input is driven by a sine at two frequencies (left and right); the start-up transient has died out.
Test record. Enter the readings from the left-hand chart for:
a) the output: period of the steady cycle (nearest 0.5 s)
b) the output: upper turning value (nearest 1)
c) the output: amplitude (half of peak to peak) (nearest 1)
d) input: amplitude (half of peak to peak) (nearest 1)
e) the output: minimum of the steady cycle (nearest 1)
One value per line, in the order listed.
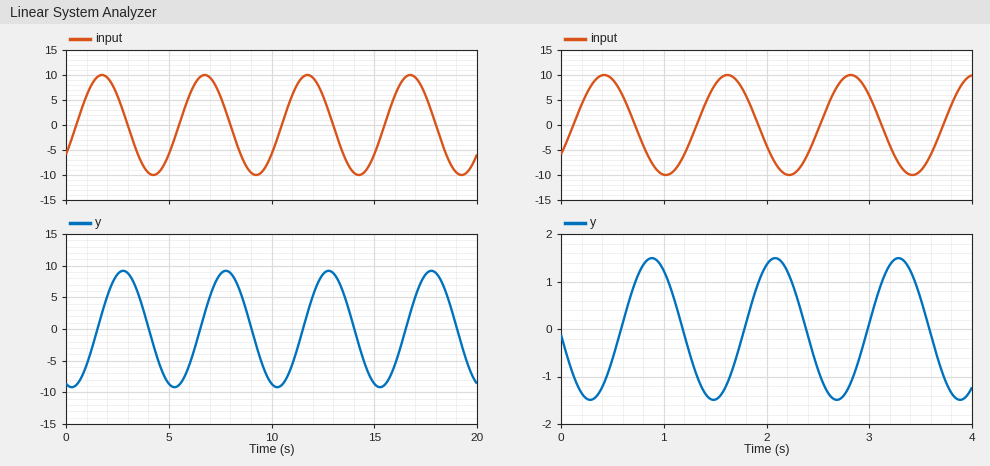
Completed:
5.0 s
9
9
10
-9
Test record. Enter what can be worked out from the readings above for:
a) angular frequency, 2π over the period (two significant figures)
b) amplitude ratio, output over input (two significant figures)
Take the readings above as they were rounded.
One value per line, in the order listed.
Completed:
1.3 rad/s
0.90
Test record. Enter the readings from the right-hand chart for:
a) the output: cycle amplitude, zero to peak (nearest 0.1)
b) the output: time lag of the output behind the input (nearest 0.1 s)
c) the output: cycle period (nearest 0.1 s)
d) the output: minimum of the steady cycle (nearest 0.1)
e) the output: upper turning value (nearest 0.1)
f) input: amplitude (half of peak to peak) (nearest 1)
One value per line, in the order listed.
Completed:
1.5
0.5 s
1.2 s
-1.5
1.5
10
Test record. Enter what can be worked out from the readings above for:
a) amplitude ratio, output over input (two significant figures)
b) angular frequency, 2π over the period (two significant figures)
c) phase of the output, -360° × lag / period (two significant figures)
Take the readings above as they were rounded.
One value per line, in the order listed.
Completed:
0.15
5.2 rad/s
-150°
